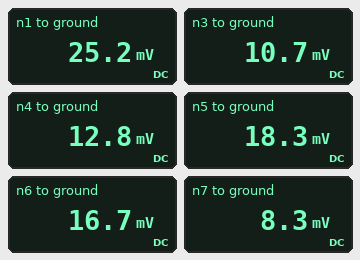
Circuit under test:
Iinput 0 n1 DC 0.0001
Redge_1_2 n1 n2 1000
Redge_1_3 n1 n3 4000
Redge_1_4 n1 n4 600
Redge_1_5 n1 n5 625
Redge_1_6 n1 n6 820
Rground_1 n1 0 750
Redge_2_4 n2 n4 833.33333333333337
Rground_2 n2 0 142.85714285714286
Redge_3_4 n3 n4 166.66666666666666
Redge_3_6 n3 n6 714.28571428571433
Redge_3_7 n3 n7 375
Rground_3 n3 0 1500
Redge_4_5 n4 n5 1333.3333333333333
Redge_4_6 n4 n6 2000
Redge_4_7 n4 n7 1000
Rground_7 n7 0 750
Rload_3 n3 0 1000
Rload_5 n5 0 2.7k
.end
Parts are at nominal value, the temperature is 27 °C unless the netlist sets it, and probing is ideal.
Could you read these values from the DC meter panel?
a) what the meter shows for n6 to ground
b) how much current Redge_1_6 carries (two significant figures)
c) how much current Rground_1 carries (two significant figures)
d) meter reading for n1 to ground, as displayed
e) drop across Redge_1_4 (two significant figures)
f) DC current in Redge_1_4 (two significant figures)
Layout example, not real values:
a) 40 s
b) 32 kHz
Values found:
a) 16.7 mV
b) 10 µA
c) 34 µA
d) 25.2 mV
e) 12 mV
f) 21 µA
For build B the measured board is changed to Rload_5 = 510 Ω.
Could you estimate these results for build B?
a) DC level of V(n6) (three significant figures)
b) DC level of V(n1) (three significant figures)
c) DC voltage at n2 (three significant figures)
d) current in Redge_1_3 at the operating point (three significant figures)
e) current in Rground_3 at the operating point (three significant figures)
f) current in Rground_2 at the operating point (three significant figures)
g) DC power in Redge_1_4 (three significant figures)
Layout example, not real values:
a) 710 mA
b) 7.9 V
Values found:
a) 14.4 mV
b) 22.2 mV
c) 3.79 mV
d) 3.33 µA
e) 5.96 µA
f) 26.5 µA
g) 229 nW
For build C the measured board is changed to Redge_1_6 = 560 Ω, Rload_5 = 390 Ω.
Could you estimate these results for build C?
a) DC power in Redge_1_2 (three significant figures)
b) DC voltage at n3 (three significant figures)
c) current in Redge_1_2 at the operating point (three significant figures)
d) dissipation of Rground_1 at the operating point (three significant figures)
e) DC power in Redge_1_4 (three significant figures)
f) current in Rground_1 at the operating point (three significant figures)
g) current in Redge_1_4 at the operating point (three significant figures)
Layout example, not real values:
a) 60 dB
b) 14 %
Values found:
a) 316 nW
b) 8.86 mV
c) 17.8 µA
d) 613 nW
e) 208 nW
f) 28.6 µA
g) 18.6 µA
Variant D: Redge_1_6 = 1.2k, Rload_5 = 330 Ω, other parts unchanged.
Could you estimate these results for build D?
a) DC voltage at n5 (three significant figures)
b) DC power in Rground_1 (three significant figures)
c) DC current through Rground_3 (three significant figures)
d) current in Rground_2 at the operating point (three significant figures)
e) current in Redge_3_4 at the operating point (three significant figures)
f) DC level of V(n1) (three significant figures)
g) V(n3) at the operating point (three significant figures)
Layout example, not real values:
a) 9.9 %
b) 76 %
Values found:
a) 7.80 mV
b) 626 nW
c) 5.47 µA
d) 25.4 µA
e) 9.17 µA
f) 21.7 mV
g) 8.20 mV
